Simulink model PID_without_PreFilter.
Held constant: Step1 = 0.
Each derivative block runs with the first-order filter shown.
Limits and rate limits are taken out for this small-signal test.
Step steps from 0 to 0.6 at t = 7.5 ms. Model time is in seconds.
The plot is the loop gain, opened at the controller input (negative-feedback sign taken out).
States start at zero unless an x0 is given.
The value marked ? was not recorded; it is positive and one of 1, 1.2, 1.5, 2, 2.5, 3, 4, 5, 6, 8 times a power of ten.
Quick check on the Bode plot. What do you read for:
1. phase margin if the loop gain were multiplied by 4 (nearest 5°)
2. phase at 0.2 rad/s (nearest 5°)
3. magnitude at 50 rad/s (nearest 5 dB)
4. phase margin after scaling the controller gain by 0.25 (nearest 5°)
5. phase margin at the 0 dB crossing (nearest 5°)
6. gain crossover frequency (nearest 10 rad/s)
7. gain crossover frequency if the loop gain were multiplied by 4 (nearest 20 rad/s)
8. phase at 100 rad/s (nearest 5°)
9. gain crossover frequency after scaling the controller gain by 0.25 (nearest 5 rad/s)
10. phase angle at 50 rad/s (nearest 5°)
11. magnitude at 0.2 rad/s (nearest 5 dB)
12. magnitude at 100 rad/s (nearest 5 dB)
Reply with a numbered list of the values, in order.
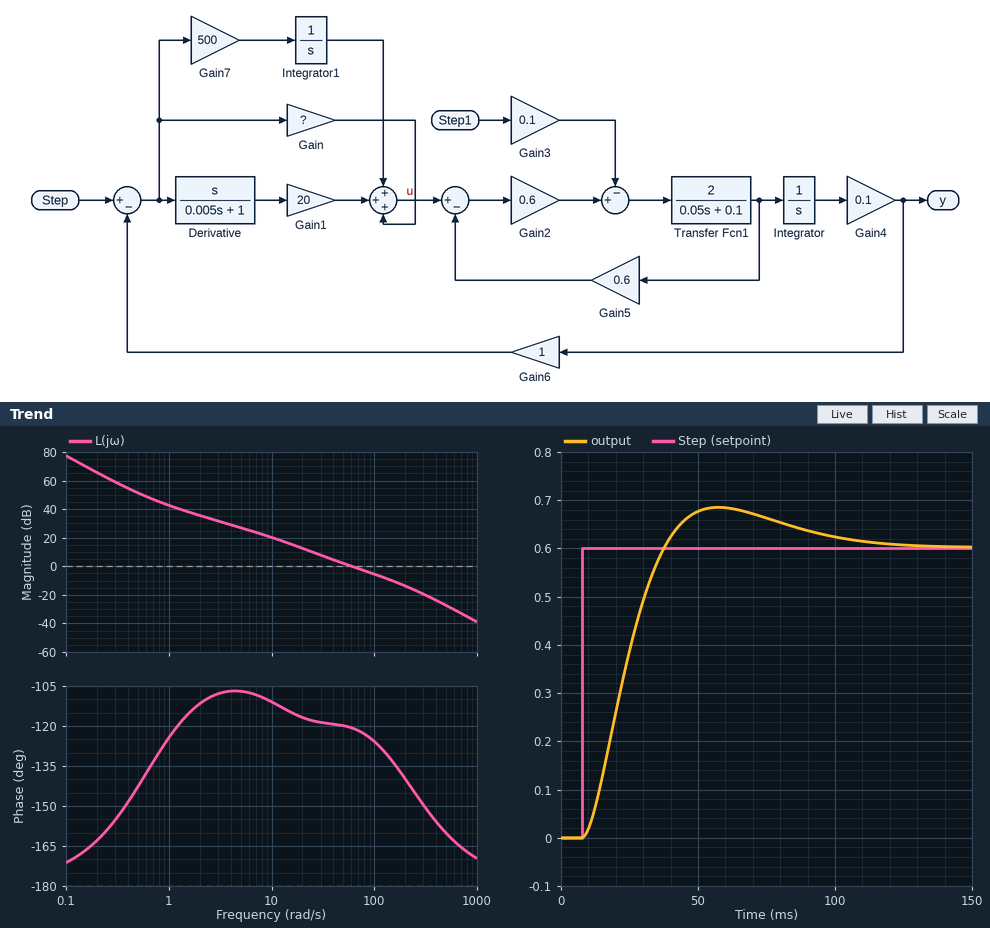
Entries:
1. 45°
2. -165°
3. 0 dB
4. 65°
5. 60°
6. 60 rad/s
7. 180 rad/s
8. -125°
9. 20 rad/s
10. -120°
11. 65 dB
12. -5 dB
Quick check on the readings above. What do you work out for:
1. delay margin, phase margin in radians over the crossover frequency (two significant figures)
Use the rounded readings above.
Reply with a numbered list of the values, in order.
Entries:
1. 0.017 s
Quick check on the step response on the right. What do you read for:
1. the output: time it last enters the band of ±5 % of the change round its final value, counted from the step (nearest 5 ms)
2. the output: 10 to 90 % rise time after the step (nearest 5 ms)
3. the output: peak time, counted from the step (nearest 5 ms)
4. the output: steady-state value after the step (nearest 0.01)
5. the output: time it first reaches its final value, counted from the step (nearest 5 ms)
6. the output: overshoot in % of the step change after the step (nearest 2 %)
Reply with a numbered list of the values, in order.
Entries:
1. 85 ms
2. 20 ms
3. 50 ms
4. 0.60
5. 30 ms
6. 14 %
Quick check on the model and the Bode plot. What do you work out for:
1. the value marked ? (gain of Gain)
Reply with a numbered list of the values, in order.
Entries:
1. 800
